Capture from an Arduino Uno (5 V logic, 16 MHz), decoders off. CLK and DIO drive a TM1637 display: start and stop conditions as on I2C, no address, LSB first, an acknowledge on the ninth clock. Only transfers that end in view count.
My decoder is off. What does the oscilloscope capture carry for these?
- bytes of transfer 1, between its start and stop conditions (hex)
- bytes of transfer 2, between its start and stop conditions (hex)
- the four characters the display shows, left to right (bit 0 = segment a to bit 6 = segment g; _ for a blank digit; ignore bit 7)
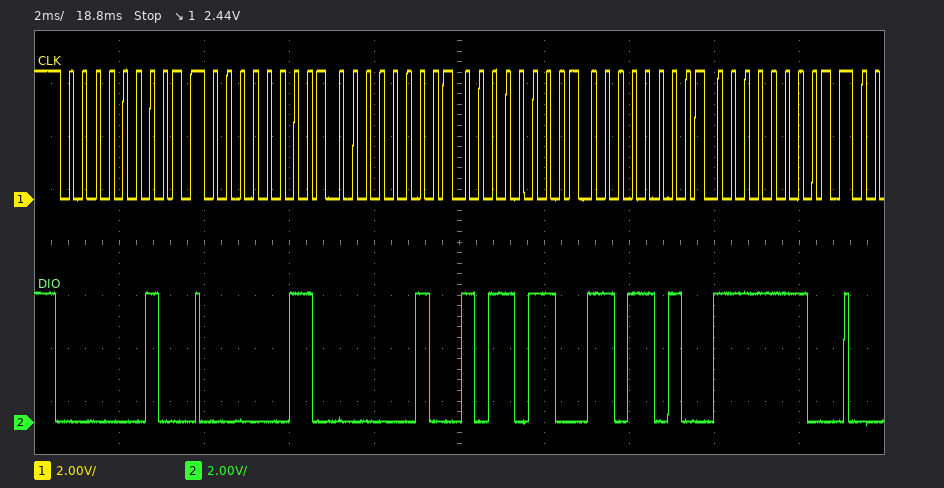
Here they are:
40
C0 40 6D 5B 7F
-528
